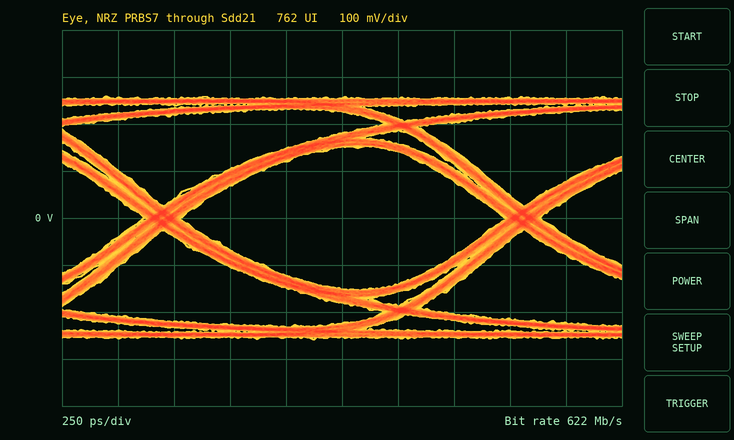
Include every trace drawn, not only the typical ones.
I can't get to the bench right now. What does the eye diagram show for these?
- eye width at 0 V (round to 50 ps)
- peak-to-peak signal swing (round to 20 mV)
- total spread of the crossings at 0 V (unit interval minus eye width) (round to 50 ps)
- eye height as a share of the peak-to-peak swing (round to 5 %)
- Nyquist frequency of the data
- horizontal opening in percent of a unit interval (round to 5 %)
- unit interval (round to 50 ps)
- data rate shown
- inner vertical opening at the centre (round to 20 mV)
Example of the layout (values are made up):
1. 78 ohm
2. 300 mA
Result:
1. 1.45 ns
2. 520 mV
3. 150 ps
4. 60 %
5. 311 MHz
6. 90 %
7. 1.60 ns
8. 622 Mb/s
9. 300 mV
